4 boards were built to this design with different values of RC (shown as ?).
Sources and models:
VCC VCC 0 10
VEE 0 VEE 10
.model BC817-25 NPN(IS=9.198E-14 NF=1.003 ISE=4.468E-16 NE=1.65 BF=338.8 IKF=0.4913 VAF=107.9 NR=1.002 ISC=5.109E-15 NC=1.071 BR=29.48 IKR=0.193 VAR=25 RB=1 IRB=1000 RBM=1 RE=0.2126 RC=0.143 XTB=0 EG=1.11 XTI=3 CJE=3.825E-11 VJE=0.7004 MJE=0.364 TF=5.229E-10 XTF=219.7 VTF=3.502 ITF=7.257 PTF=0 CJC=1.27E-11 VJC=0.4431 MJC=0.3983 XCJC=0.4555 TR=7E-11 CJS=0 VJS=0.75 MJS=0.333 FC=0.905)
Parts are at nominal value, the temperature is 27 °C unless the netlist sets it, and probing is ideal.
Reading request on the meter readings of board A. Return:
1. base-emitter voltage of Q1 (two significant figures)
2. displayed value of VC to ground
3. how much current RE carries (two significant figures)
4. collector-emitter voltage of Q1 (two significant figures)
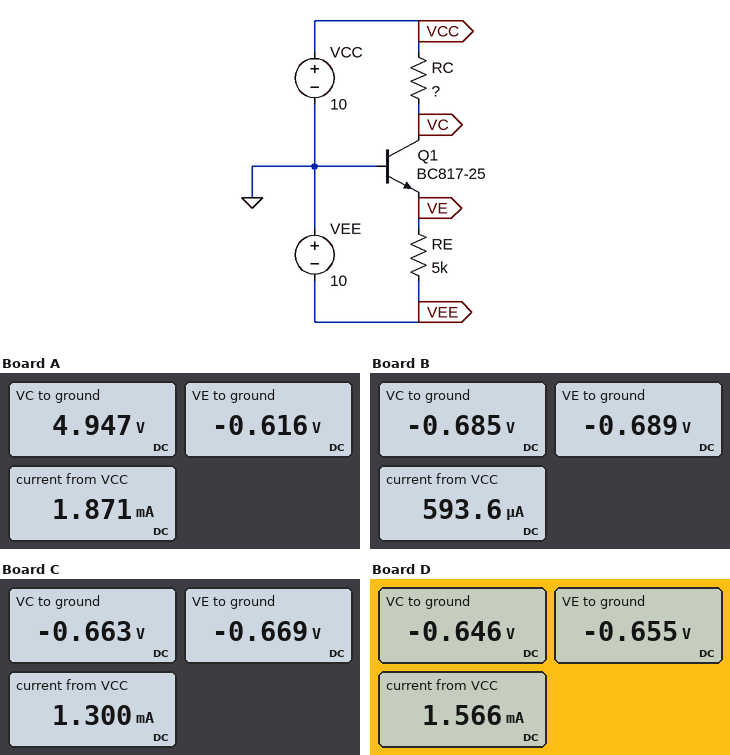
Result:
620 mV
4.947 V
1.9 mA
5.6 V
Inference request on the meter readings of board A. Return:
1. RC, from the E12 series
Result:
2.7 kΩ
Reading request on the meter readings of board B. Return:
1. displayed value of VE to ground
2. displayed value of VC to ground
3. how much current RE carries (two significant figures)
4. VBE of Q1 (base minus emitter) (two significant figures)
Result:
-0.689 V
-0.685 V
1.9 mA
690 mV
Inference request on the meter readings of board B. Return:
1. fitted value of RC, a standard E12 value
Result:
18 kΩ
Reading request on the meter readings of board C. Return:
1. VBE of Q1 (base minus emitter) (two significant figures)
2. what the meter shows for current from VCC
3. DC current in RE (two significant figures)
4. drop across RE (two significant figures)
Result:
670 mV
1.300 mA
1.9 mA
9.3 V
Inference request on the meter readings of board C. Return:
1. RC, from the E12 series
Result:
8.2 kΩ
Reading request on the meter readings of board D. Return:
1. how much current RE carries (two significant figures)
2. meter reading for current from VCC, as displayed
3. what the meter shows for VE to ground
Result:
1.9 mA
1.566 mA
-0.655 V
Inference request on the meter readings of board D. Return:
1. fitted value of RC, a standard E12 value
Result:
6.8 kΩ
